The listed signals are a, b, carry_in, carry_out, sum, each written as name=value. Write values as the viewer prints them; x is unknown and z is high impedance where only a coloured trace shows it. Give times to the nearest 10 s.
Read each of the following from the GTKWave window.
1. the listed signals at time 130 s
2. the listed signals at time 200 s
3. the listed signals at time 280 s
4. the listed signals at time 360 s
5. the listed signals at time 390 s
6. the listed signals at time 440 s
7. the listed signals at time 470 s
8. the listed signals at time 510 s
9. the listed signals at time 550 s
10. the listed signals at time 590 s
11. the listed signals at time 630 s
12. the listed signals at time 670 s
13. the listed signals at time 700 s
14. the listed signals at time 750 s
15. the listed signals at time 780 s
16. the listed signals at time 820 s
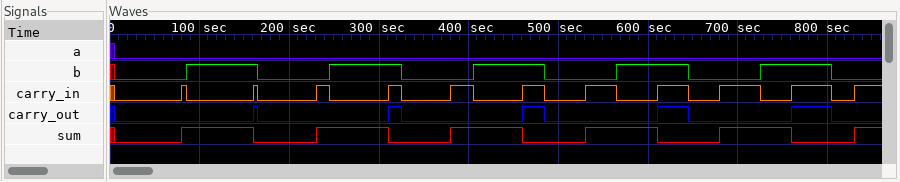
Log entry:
a=0, b=1, carry_in=0, carry_out=0, sum=1
a=0, b=0, carry_in=0, carry_out=0, sum=0
a=0, b=1, carry_in=0, carry_out=0, sum=1
a=0, b=0, carry_in=0, carry_out=0, sum=0
a=0, b=0, carry_in=1, carry_out=0, sum=1
a=0, b=1, carry_in=0, carry_out=0, sum=1
a=0, b=1, carry_in=1, carry_out=1, sum=0
a=0, b=0, carry_in=0, carry_out=0, sum=0
a=0, b=0, carry_in=1, carry_out=0, sum=1
a=0, b=1, carry_in=0, carry_out=0, sum=1
a=0, b=1, carry_in=1, carry_out=1, sum=0
a=0, b=0, carry_in=0, carry_out=0, sum=0
a=0, b=0, carry_in=1, carry_out=0, sum=1
a=0, b=1, carry_in=0, carry_out=0, sum=1
a=0, b=1, carry_in=1, carry_out=1, sum=0
a=0, b=0, carry_in=0, carry_out=0, sum=0
